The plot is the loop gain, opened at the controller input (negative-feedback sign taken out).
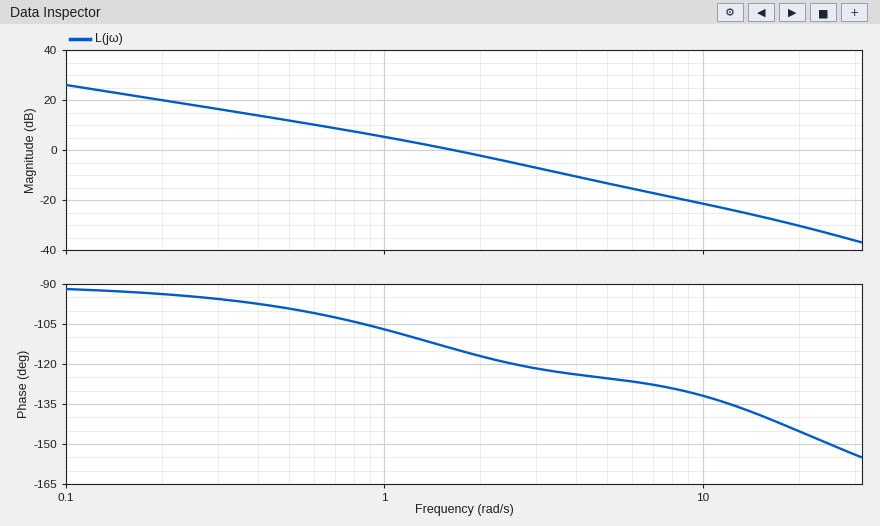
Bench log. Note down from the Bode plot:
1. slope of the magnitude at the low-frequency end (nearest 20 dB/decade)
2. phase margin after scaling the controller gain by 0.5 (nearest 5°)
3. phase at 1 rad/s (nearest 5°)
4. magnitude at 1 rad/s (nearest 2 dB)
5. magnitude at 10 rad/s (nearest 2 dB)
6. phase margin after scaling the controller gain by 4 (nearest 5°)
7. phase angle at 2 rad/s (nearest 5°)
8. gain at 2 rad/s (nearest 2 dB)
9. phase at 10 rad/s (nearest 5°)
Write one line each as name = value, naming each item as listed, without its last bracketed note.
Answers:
slope of the magnitude at the low-frequency end = -20 dB/decade
phase margin after scaling the controller gain by 0.5 = 75°
phase at 1 rad/s = -105°
magnitude at 1 rad/s = 6 dB
magnitude at 10 rad/s = -22 dB
phase margin after scaling the controller gain by 4 = 55°
phase angle at 2 rad/s = -115°
gain at 2 rad/s = -2 dB
phase at 10 rad/s = -130°
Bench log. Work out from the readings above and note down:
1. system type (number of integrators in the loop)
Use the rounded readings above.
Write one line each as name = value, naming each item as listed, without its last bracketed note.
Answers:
system type = 1
